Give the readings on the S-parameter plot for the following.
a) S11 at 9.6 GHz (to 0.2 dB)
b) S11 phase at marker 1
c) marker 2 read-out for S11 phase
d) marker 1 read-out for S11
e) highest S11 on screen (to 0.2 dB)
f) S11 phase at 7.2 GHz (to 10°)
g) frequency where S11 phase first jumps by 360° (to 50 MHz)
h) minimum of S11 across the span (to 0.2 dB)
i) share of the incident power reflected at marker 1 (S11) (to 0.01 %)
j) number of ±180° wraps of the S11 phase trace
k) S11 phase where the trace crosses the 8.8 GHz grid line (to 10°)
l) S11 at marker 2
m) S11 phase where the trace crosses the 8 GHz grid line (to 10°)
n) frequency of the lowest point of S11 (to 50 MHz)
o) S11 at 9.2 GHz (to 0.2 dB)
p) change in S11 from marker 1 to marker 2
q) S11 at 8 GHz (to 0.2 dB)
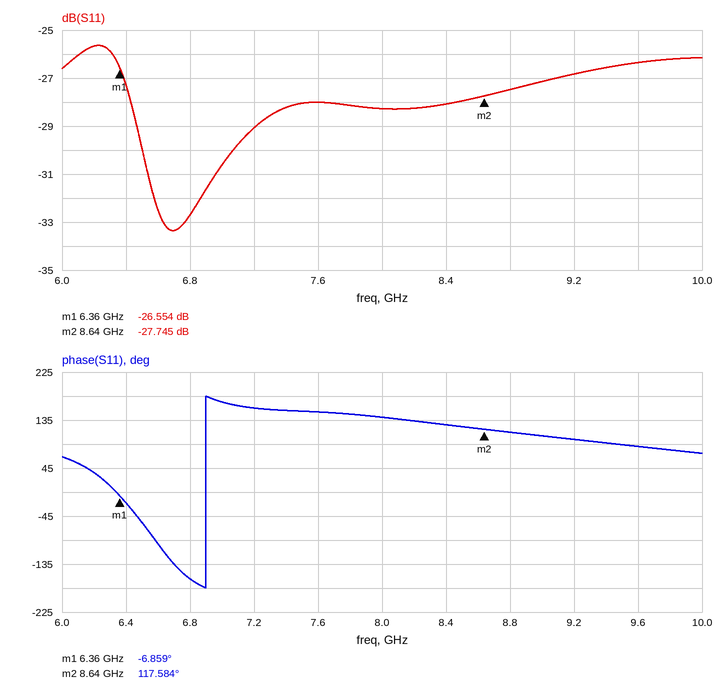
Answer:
-26.4 dB
-6.859°
117.584°
-26.554 dB
-25.6 dB
160°
6.90 GHz
-33.4 dB
0.22 %
1
110°
-27.745 dB
140°
6.70 GHz
-26.8 dB
-1.191 dB
-28.2 dB
